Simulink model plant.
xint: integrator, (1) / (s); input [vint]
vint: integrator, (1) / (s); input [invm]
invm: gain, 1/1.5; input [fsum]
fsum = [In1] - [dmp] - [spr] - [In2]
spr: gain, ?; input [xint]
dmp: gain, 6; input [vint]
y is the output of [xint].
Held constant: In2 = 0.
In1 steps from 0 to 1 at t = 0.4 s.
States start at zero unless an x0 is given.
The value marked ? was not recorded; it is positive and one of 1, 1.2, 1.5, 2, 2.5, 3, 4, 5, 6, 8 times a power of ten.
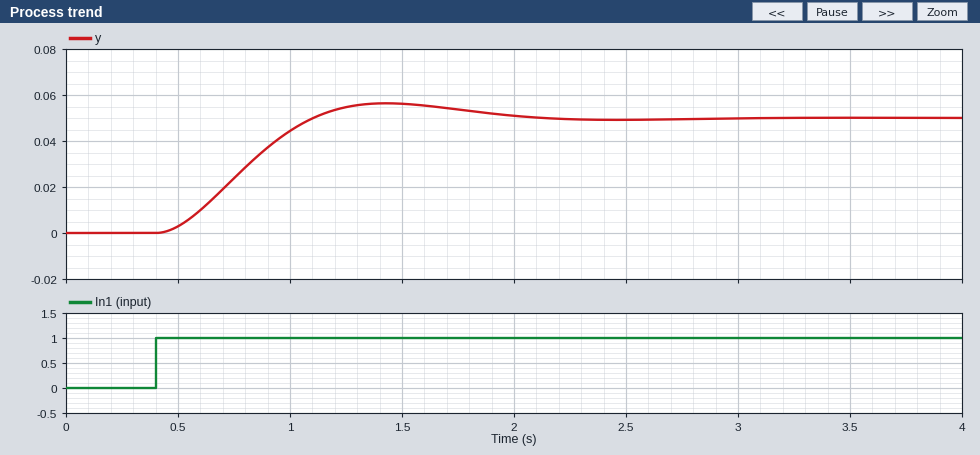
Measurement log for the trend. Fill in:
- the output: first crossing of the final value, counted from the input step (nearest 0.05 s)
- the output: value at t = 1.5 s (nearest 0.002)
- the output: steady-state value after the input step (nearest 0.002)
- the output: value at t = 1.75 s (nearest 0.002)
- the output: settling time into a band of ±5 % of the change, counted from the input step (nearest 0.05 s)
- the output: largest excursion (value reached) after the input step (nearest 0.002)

0.70 s
0.056
0.050
0.054
1.45 s
0.056
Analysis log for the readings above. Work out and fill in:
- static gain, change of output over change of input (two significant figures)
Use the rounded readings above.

0.050
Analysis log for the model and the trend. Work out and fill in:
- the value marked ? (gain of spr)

20
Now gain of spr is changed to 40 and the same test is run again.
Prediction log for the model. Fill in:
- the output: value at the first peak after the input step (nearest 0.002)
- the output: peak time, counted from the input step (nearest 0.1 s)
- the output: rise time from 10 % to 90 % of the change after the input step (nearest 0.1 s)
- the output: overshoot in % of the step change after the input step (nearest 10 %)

0.032
0.7 s
0.3 s
30 %
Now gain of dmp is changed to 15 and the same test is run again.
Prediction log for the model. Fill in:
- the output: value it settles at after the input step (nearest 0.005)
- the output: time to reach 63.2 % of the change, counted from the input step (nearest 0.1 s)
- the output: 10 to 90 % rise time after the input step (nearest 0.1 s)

0.050
0.8 s
1.4 s
